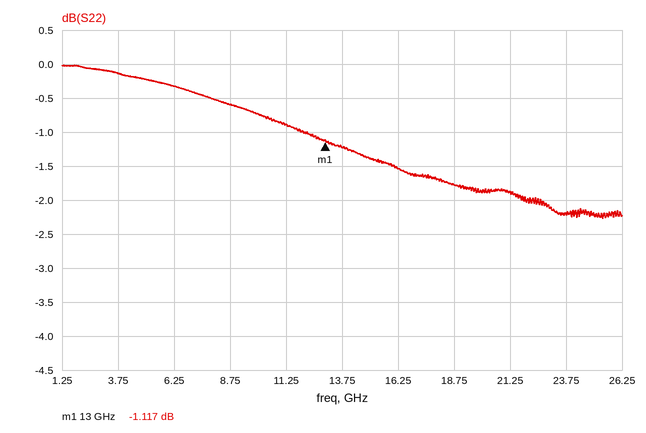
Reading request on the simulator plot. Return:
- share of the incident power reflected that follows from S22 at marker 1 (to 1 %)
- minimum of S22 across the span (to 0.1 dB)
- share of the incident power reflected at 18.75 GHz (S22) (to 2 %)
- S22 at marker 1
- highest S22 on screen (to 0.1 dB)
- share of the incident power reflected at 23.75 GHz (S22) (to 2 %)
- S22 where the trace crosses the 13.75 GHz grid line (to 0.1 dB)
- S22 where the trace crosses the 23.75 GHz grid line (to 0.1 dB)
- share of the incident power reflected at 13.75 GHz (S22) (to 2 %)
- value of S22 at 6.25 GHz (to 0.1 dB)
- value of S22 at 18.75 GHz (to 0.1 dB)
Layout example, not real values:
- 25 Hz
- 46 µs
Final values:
- 77 %
- -2.3 dB
- 66 %
- -1.117 dB
- 0.0 dB
- 60 %
- -1.2 dB
- -2.2 dB
- 76 %
- -0.3 dB
- -1.8 dB
